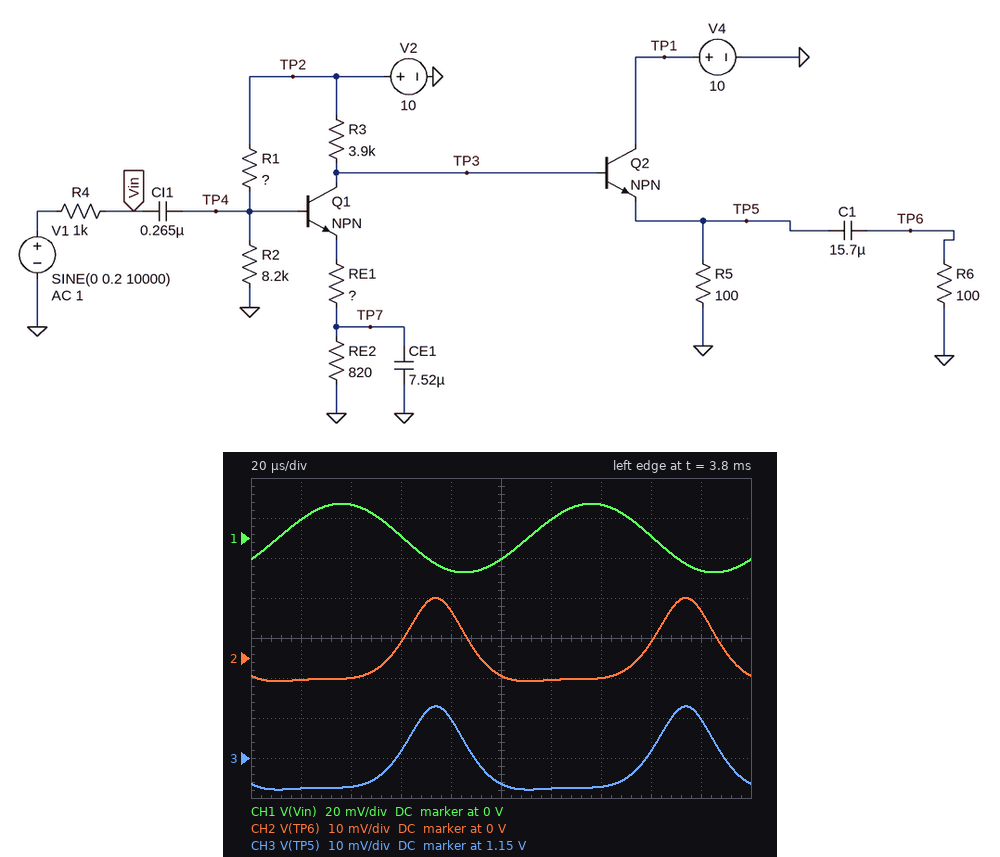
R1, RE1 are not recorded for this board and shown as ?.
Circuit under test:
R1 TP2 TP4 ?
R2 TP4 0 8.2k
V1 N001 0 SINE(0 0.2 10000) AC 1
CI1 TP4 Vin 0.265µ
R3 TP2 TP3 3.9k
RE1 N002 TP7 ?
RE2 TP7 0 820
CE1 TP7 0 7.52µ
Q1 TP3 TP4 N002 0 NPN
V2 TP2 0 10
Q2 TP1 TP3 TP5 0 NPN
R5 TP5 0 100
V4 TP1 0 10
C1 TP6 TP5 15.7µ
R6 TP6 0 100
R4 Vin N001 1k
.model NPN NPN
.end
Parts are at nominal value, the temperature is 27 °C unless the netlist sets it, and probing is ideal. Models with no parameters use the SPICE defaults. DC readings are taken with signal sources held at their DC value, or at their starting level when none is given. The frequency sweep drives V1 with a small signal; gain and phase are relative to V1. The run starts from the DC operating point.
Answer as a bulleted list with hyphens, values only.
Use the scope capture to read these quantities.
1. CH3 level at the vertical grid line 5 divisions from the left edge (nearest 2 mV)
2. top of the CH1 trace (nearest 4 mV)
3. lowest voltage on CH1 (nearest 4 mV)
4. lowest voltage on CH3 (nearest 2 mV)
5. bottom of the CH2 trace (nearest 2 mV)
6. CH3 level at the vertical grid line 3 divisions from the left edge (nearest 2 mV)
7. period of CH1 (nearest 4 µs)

- 1.144 V
- 16 mV
- -16 mV
- 1.142 V
- -6 mV
- 1.152 V
- 100 µs
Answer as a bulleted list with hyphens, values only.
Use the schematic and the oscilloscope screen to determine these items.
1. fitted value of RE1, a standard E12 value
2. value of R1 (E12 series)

- 47 Ω
- 12 kΩ
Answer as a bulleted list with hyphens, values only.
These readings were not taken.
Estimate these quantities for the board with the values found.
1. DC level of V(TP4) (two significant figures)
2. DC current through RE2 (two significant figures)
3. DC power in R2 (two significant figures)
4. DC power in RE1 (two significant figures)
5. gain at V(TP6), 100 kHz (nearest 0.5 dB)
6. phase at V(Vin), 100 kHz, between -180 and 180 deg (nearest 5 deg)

- 2.7 V
- 2.2 mA
- 900 µW
- 230 µW
- -31.0 dB
- -5 deg
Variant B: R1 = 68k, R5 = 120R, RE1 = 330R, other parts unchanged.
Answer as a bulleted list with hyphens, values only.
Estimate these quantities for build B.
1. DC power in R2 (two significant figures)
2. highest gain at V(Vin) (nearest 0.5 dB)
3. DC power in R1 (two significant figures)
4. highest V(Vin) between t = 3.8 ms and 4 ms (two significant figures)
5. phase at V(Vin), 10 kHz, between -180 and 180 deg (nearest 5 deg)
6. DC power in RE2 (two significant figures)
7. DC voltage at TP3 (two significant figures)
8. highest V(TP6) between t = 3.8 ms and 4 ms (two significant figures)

- 140 µW
- 0 dB
- 1.2 mW
- 170 mV
- 0 deg
- 62 µW
- 7.0 V
- 650 mV
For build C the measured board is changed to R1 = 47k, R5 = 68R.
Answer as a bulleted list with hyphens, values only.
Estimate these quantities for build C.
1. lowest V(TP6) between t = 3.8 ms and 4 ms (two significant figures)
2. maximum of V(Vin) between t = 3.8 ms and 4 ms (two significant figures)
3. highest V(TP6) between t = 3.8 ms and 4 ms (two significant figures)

- -2.3 V
- 150 mV
- 1.5 V
